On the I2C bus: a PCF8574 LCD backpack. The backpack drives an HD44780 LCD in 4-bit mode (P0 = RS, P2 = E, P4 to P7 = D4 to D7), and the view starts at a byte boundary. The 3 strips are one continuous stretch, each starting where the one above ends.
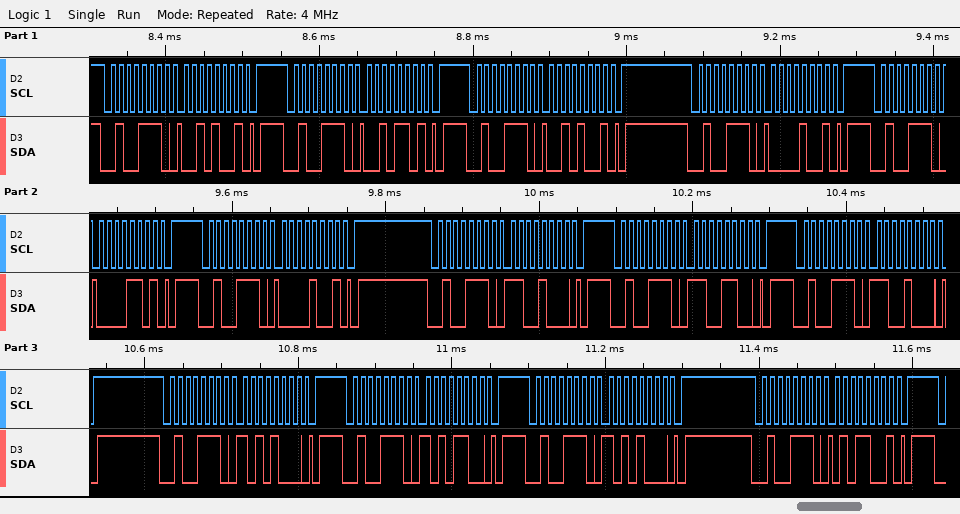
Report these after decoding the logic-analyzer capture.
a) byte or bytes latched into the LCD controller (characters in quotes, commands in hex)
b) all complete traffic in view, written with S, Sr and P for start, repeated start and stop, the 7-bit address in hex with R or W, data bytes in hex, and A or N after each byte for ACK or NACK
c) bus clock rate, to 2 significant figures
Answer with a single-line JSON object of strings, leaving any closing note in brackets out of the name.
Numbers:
{"byte or bytes latched into the LCD controller": "' ' 0xCA", "all complete traffic in view, written with S, Sr and P for start, repeated start and stop, the 7-bit address in hex with R or W, data bytes in hex, and A or N after each byte for ACK or NACK": "S 27W A 29 A P S 27W A 2D A P S 27W A 29 A P S 27W A 09 A P S 27W A 0D A P S 27W A 09 A P S 27W A C8 A P S 27W A CC A P S 27W A C8 A P S 27W A A8 A P S 27W A AC A P S 27W A A8 A P S 27W A 59 A P", "bus clock rate, to 2 significant figures": "100 kHz"}
